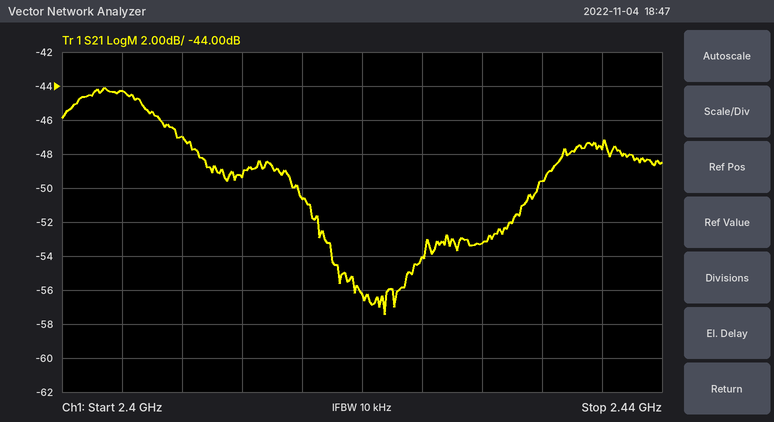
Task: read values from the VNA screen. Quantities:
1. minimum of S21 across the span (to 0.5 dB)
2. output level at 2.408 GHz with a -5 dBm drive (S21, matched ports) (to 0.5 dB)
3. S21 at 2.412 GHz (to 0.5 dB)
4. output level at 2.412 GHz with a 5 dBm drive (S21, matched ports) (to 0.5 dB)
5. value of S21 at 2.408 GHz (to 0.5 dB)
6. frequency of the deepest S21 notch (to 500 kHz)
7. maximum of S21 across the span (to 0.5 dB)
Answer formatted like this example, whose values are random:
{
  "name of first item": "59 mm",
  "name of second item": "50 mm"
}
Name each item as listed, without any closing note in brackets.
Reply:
{
  "minimum of S21 across the span": "-57.5 dB",
  "output level at 2.408 GHz with a -5 dBm drive (S21, matched ports)": "-52.0 dBm",
  "S21 at 2.412 GHz": "-49.5 dB",
  "output level at 2.412 GHz with a 5 dBm drive (S21, matched ports)": "-44.5 dBm",
  "value of S21 at 2.408 GHz": "-47.0 dB",
  "frequency of the deepest S21 notch": "2.4215 GHz",
  "maximum of S21 across the span": "-44.0 dB"
}
